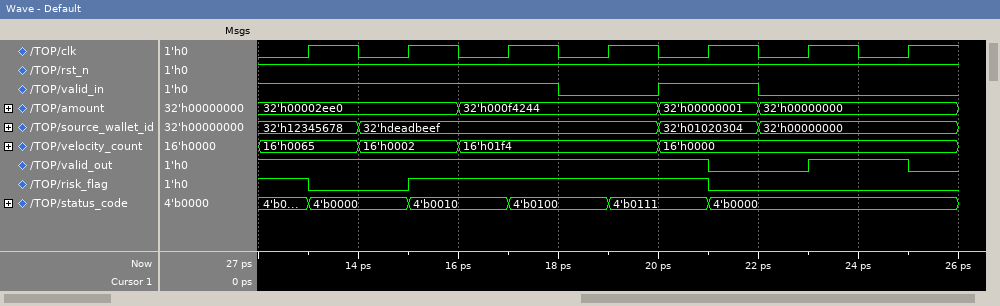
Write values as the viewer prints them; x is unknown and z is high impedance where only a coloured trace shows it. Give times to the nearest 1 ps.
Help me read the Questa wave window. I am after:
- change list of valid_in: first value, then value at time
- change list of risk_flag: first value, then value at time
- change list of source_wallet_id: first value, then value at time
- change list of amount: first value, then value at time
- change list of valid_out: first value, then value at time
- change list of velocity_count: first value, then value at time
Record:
1, 0 at 18 ps, 1 at 20 ps, 0 at 22 ps
1, 0 at 13 ps, 1 at 15 ps, 0 at 21 ps
32'h12345678, 32'hdeadbeef at 14 ps, 32'h01020304 at 20 ps, 32'h00000000 at 22 ps
32'h00002ee0, 32'h000f4244 at 16 ps, 32'h00000001 at 20 ps, 32'h00000000 at 22 ps
1, 0 at 21 ps, 1 at 23 ps, 0 at 25 ps
16'h0065, 16'h0002 at 14 ps, 16'h01f4 at 16 ps, 16'h0000 at 20 ps
